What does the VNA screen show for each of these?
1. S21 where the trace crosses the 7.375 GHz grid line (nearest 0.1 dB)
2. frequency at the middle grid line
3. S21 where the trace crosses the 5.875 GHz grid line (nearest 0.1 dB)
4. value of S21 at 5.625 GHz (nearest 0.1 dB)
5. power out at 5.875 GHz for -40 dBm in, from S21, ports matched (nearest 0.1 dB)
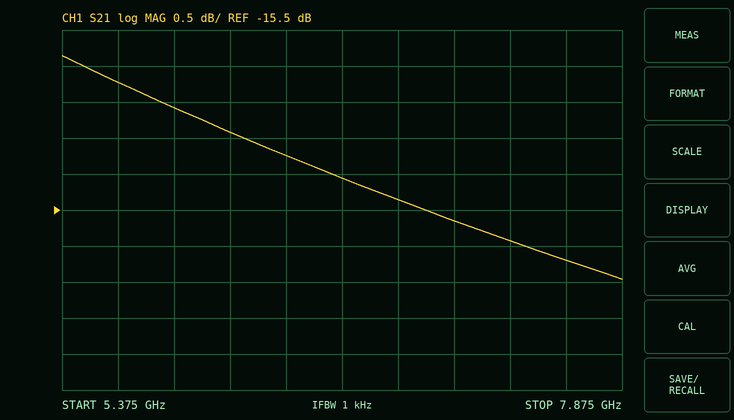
-15.9 dB
6.625 GHz
-14.1 dB
-13.7 dB
-54.1 dBm
